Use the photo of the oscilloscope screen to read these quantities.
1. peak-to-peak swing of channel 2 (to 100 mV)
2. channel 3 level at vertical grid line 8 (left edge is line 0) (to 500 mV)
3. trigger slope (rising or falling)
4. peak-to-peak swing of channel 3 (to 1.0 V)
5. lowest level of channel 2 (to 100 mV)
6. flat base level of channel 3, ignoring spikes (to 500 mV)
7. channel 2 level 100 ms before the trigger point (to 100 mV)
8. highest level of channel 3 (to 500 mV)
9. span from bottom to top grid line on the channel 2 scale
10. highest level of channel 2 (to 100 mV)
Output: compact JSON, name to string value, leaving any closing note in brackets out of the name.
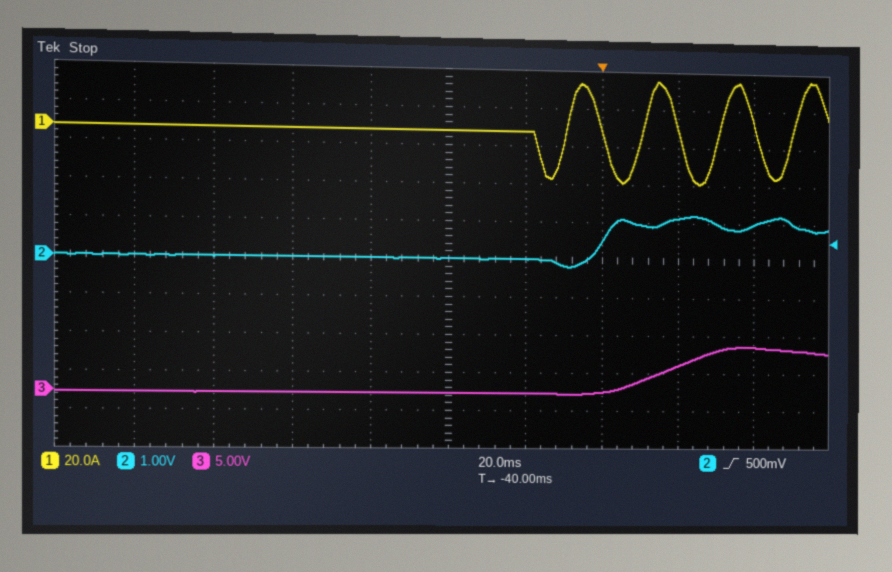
{"peak-to-peak swing of channel 2": "1.4 V", "channel 3 level at vertical grid line 8 (left edge is line 0)": "3.5 V", "trigger slope": "rising", "peak-to-peak swing of channel 3": "6.0 V", "lowest level of channel 2": "-200 mV", "flat base level of channel 3, ignoring spikes": "0.0 V", "channel 2 level 100 ms before the trigger point": "0.0 V", "highest level of channel 3": "6.0 V", "span from bottom to top grid line on the channel 2 scale": "10 V", "highest level of channel 2": "1.2 V"}
